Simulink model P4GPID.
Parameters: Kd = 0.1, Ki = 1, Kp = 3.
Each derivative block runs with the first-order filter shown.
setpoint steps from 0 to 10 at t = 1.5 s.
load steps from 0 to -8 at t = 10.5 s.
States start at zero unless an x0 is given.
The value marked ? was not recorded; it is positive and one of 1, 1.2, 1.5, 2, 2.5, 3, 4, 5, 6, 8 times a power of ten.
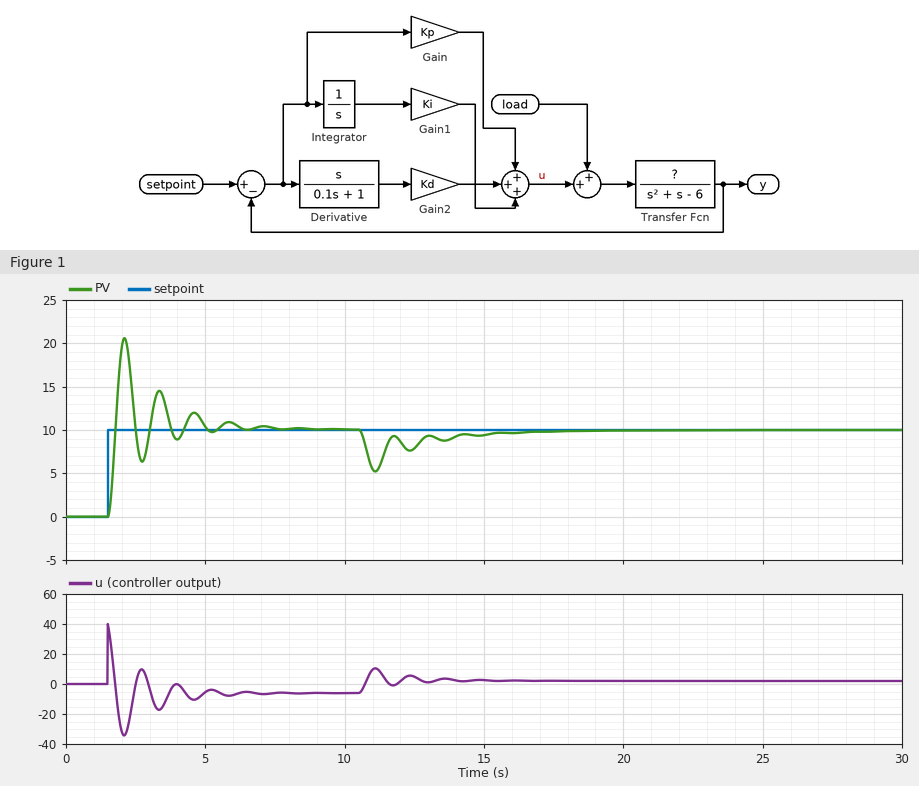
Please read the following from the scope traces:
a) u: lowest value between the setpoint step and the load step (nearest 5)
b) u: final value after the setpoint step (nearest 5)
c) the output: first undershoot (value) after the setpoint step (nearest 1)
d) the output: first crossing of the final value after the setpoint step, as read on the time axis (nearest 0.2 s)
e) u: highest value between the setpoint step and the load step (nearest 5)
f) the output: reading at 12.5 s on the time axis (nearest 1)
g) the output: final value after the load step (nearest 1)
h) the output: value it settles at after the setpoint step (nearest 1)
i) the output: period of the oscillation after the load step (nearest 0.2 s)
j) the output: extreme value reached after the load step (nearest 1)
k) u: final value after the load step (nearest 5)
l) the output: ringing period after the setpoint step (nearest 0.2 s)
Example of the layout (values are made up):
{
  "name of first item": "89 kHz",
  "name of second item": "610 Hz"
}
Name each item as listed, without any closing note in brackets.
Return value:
{
  "u: lowest value between the setpoint step and the load step": "-35",
  "u: final value after the setpoint step": "-5",
  "the output: first undershoot (value) after the setpoint step": "6",
  "the output: first crossing of the final value after the setpoint step, as read on the time axis": "1.8 s",
  "u: highest value between the setpoint step and the load step": "40",
  "the output: reading at 12.5 s on the time axis": "8",
  "the output: final value after the load step": "10",
  "the output: value it settles at after the setpoint step": "10",
  "the output: period of the oscillation after the load step": "1.2 s",
  "the output: extreme value reached after the load step": "5",
  "u: final value after the load step": "0",
  "the output: ringing period after the setpoint step": "1.2 s"
}
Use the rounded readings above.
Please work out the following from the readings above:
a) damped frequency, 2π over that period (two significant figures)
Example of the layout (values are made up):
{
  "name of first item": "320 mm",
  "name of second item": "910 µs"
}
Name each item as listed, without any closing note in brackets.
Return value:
{
  "damped frequency, 2π over that period": "5.2 rad/s"
}
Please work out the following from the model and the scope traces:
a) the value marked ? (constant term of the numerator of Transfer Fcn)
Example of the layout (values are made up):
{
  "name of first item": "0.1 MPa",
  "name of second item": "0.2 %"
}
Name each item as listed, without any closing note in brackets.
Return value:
{
  "the value marked ?": "10"
}
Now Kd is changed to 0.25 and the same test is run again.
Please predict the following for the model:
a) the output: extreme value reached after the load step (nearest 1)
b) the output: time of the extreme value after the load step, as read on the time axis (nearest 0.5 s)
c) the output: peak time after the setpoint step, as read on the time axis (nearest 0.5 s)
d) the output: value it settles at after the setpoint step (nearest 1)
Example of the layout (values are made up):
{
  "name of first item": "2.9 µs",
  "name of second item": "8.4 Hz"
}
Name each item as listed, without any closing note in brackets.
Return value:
{
  "the output: extreme value reached after the load step": "6",
  "the output: time of the extreme value after the load step, as read on the time axis": "11.0 s",
  "the output: peak time after the setpoint step, as read on the time axis": "2.0 s",
  "the output: value it settles at after the setpoint step": "10"
}
